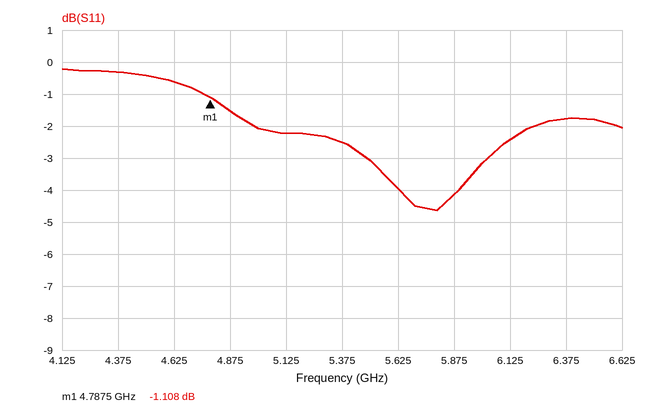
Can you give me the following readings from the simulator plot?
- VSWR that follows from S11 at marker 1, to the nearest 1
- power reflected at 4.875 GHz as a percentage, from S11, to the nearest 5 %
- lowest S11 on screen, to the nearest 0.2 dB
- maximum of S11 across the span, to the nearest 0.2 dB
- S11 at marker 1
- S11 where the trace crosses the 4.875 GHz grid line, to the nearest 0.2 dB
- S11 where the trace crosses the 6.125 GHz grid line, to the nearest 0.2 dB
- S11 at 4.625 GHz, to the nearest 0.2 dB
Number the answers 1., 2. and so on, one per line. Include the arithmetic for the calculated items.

1. (1 + 0.8802)/(1 − 0.8802) ≈ 16
2. 10^(-1.6/10) ≈ 69.2 %, so 70 % to the nearest 5 %
3. -4.6 dB
4. -0.2 dB
5. -1.108 dB
6. -1.6 dB
7. -2.4 dB
8. -0.6 dB
